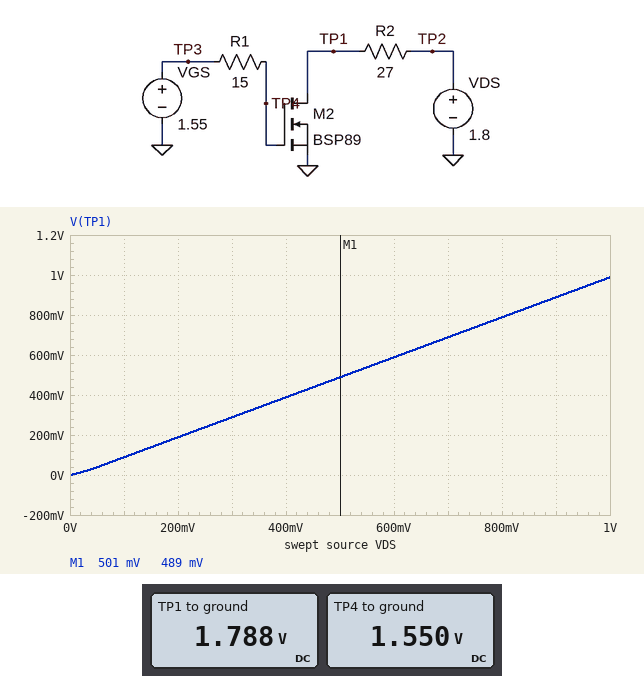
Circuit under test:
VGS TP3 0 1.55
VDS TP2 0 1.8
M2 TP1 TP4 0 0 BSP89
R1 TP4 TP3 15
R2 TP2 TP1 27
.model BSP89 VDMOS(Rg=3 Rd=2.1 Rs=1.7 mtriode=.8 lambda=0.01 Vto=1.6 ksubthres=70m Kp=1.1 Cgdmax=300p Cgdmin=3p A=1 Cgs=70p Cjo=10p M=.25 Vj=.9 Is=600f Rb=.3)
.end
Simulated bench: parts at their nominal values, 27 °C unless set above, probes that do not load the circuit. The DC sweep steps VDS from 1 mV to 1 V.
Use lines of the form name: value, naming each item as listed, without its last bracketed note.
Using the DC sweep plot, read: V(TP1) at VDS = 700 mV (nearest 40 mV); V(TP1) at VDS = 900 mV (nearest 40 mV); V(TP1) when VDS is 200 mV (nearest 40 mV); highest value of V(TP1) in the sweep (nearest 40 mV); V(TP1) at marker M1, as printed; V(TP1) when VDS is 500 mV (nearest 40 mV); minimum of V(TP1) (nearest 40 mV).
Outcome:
V(TP1) at VDS = 700 mV: 680 mV
V(TP1) at VDS = 900 mV: 880 mV
V(TP1) when VDS is 200 mV: 200 mV
highest value of V(TP1) in the sweep: 1.00 V
V(TP1) at marker M1, as printed: 489 mV
V(TP1) when VDS is 500 mV: 480 mV
minimum of V(TP1): 0 V
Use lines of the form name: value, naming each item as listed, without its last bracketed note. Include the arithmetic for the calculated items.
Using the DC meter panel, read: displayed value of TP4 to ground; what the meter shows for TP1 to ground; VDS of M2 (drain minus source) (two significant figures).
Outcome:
displayed value of TP4 to ground: 1.550 V
what the meter shows for TP1 to ground: 1.788 V
VDS of M2 (drain minus source): 1.788 V = 1.8 V
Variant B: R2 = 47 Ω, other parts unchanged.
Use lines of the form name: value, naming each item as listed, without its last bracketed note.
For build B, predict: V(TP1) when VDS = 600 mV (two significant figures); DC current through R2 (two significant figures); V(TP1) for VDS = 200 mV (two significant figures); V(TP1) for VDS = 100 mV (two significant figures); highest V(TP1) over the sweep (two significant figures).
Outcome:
V(TP1) when VDS = 600 mV: 580 mV
DC current through R2: 430 µA
V(TP1) for VDS = 200 mV: 180 mV
V(TP1) for VDS = 100 mV: 80 mV
highest V(TP1) over the sweep: 980 mV
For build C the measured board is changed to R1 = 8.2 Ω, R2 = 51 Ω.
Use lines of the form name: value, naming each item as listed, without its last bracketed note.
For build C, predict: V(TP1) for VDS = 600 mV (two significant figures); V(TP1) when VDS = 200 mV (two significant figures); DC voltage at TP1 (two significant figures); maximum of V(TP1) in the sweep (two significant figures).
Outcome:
V(TP1) for VDS = 600 mV: 580 mV
V(TP1) when VDS = 200 mV: 180 mV
DC voltage at TP1: 1.8 V
maximum of V(TP1) in the sweep: 980 mV
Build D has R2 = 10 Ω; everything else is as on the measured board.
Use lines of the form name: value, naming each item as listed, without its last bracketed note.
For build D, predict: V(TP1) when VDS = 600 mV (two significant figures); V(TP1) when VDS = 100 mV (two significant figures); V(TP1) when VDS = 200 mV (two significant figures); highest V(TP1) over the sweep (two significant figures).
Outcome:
V(TP1) when VDS = 600 mV: 600 mV
V(TP1) when VDS = 100 mV: 96 mV
V(TP1) when VDS = 200 mV: 200 mV
highest V(TP1) over the sweep: 1.0 V
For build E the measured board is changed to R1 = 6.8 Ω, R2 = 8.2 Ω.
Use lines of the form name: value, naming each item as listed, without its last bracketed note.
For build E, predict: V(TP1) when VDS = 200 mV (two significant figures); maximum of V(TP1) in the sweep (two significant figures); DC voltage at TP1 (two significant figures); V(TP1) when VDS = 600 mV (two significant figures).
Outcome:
V(TP1) when VDS = 200 mV: 200 mV
maximum of V(TP1) in the sweep: 1.0 V
DC voltage at TP1: 1.8 V
V(TP1) when VDS = 600 mV: 600 mV
